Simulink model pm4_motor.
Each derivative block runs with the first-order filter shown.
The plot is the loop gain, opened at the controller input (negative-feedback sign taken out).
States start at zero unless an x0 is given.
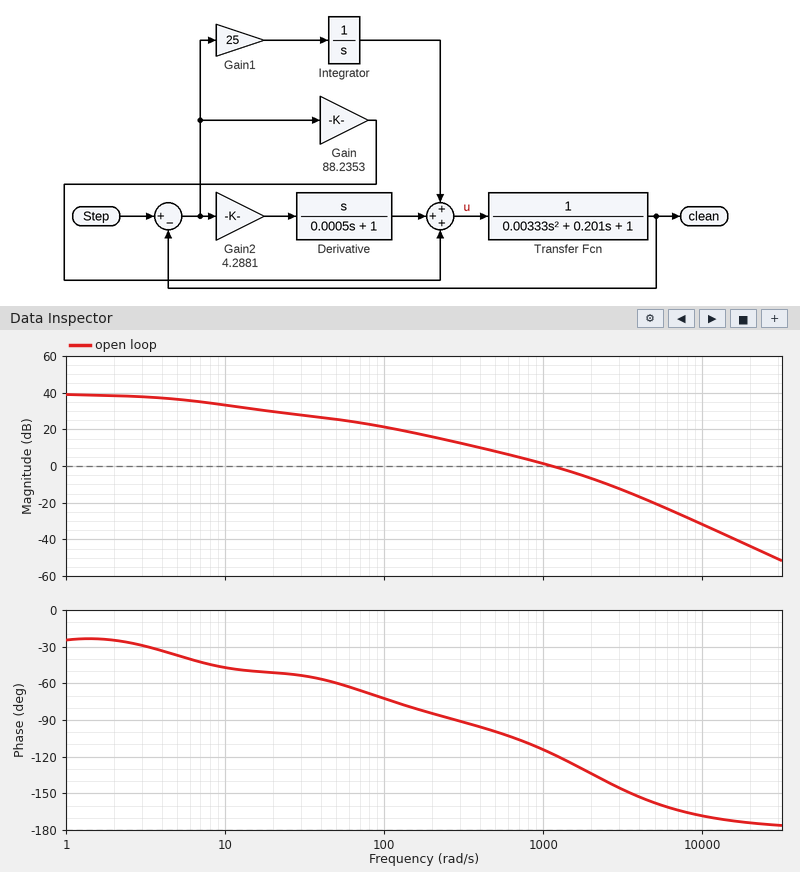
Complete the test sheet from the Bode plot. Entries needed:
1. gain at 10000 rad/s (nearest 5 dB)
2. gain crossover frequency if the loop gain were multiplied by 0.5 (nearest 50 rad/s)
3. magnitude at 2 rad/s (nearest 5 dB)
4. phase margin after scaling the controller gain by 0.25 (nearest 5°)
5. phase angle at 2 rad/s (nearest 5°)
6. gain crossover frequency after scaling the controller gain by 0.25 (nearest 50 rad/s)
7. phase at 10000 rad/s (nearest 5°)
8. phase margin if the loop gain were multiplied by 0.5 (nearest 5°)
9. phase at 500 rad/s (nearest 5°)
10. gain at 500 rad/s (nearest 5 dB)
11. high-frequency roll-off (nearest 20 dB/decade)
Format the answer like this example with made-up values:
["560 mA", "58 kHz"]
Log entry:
["-30 dB", "600 rad/s", "40 dB", "90°", "-25°", "300 rad/s", "-170°", "75°", "-100°", "10 dB", "-40 dB/decade"]
